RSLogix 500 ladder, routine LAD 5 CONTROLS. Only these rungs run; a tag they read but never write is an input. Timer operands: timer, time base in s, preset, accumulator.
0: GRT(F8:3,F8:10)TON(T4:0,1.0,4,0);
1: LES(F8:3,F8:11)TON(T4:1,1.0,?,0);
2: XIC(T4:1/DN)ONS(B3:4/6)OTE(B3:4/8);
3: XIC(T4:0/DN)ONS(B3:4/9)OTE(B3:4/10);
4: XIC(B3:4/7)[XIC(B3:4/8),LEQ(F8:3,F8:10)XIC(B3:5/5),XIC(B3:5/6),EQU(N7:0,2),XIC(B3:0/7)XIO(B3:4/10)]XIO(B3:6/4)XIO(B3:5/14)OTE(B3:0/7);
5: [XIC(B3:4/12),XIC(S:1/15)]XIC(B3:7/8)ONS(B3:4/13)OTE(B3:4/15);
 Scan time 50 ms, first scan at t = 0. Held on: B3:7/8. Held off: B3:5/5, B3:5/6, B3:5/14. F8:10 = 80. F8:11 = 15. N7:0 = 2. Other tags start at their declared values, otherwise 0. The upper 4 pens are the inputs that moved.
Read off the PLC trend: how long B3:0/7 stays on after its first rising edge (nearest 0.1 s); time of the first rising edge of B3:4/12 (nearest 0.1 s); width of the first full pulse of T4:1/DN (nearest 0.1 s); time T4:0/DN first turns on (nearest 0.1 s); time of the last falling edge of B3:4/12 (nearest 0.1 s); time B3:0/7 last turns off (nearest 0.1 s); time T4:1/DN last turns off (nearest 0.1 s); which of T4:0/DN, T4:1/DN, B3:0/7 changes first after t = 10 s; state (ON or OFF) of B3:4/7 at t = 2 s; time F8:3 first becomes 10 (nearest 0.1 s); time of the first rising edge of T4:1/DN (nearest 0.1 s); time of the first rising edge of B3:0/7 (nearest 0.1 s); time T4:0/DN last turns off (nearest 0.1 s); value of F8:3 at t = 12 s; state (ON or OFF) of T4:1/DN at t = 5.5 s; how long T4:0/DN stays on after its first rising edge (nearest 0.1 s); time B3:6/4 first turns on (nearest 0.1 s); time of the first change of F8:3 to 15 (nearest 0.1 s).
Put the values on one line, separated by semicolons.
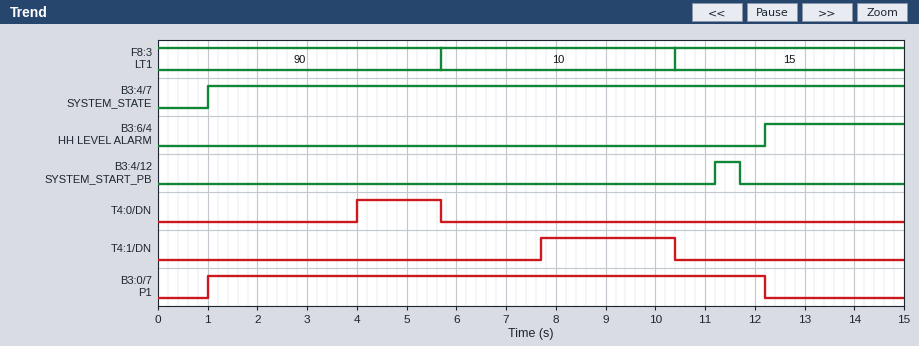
11.2 s; 11.2 s; 2.7 s; 4.0 s; 11.7 s; 12.2 s; 10.4 s; T4:1/DN; ON; 5.7 s; 7.7 s; 1.0 s; 5.7 s; 15; OFF; 1.7 s; 12.2 s; 10.4 s
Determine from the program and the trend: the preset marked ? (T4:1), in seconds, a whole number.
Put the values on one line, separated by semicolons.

2 s
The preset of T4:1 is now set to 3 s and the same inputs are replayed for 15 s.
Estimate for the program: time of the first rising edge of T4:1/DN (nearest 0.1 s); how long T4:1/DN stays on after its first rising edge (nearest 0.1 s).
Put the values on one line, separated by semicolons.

8.7 s; 1.7 s
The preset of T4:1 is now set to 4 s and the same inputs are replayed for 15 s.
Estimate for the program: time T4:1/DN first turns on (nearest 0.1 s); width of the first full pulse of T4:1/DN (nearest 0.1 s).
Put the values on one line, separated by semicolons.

9.7 s; 0.7 s
